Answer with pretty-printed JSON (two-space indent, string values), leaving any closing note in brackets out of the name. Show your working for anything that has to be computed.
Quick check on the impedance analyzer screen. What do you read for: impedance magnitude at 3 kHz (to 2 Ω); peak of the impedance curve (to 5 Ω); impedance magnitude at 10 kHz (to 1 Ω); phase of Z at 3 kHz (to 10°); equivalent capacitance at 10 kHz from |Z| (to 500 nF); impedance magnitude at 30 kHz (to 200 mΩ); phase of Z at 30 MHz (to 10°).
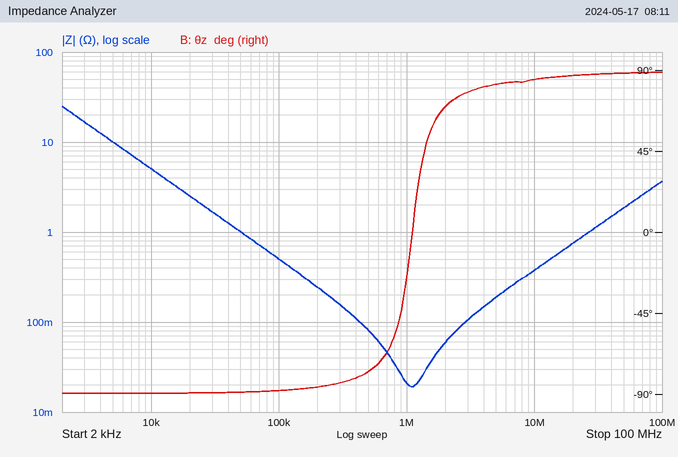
{
  "impedance magnitude at 3 kHz": "16 Ω",
  "peak of the impedance curve": "25 Ω",
  "impedance magnitude at 10 kHz": "5 Ω",
  "phase of Z at 3 kHz": "-90°",
  "equivalent capacitance at 10 kHz from |Z|": "C = 1/(2π × 10 kHz × 5 Ω) ≈ 3.18 µF, so 3.0 µF to the nearest 500 nF",
  "impedance magnitude at 30 kHz": "1.6 Ω",
  "phase of Z at 30 MHz": "90°"
}
